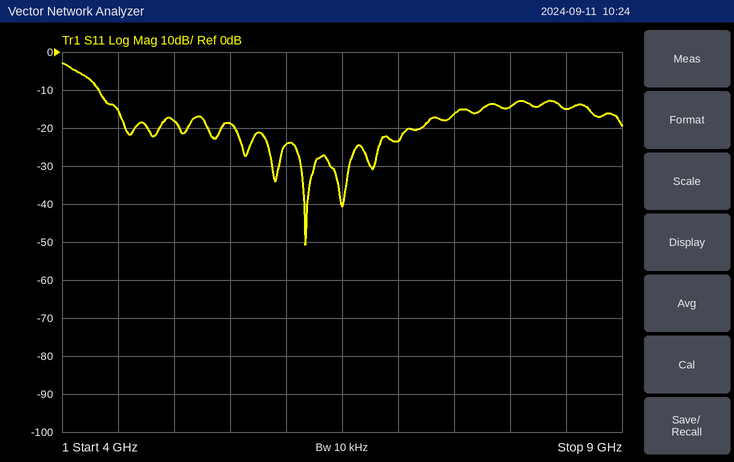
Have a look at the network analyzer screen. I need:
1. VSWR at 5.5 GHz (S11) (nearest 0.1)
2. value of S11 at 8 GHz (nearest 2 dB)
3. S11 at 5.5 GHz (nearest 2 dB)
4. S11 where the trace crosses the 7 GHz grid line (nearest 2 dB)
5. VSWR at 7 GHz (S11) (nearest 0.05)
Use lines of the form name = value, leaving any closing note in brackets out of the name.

VSWR at 5.5 GHz (S11) = 1.3
value of S11 at 8 GHz = -14 dB
S11 at 5.5 GHz = -18 dB
S11 where the trace crosses the 7 GHz grid line = -24 dB
VSWR at 7 GHz (S11) = 1.15
